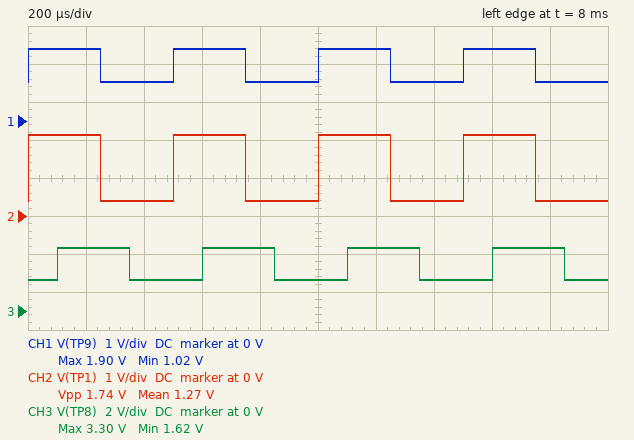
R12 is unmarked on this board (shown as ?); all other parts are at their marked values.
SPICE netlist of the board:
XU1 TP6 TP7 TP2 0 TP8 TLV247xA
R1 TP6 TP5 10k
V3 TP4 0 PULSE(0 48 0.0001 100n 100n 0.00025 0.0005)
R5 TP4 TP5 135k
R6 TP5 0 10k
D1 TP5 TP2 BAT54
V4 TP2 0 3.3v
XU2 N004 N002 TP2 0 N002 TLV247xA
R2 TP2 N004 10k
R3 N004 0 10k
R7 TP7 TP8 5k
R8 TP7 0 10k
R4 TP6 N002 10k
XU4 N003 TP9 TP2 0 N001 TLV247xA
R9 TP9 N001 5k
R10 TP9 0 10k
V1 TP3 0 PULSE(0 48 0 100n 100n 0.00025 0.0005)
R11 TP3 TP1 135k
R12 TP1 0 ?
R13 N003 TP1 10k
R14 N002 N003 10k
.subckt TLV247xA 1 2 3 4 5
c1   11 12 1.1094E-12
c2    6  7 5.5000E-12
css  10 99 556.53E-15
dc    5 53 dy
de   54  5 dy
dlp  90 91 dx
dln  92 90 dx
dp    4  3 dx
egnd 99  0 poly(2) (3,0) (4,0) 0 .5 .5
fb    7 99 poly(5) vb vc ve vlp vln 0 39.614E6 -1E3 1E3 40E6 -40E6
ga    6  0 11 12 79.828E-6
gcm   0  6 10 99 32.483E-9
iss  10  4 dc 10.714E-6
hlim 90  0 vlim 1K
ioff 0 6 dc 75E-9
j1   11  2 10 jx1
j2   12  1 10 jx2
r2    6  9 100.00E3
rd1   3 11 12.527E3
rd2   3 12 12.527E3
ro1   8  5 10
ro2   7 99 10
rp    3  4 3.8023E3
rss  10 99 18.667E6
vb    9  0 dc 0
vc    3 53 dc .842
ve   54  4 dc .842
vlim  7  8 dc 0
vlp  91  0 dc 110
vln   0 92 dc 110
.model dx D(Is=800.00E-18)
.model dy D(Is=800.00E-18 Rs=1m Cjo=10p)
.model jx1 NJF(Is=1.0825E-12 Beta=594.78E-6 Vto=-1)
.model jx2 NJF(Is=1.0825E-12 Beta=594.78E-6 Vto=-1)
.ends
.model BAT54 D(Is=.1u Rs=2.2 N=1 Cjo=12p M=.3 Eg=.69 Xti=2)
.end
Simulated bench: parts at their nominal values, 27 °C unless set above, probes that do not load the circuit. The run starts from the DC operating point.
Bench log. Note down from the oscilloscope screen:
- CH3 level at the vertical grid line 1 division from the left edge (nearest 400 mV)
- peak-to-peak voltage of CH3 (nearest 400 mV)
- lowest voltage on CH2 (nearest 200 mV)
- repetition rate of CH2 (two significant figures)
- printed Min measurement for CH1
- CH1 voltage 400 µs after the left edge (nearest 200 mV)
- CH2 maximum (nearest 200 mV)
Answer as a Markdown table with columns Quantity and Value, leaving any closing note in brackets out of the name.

| Quantity | Value |
|---|---|
| CH3 level at the vertical grid line 1 division from the left edge | 3.2 V |
| peak-to-peak voltage of CH3 | 1.6 V |
| lowest voltage on CH2 | 400 mV |
| repetition rate of CH2 | 2.0 kHz |
| printed Min measurement for CH1 | 1.02 V |
| CH1 voltage 400 µs after the left edge | 1.0 V |
| CH2 maximum | 2.2 V |
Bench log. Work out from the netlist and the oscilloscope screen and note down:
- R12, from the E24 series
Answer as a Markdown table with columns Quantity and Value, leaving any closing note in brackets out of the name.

| Quantity | Value |
|---|---|
| R12, from the E24 series | 6.8 kΩ |
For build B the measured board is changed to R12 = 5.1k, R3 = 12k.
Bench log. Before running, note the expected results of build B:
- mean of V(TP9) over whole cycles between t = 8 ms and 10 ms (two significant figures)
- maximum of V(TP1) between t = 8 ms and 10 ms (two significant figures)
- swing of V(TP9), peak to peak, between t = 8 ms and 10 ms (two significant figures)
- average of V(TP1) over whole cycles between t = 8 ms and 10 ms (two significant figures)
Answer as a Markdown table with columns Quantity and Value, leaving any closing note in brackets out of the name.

| Quantity | Value |
|---|---|
| mean of V(TP9) over whole cycles between t = 8 ms and 10 ms | 1.4 V |
| maximum of V(TP1) between t = 8 ms and 10 ms | 1.8 V |
| swing of V(TP9), peak to peak, between t = 8 ms and 10 ms | 700 mV |
| average of V(TP1) over whole cycles between t = 8 ms and 10 ms | 1.1 V |
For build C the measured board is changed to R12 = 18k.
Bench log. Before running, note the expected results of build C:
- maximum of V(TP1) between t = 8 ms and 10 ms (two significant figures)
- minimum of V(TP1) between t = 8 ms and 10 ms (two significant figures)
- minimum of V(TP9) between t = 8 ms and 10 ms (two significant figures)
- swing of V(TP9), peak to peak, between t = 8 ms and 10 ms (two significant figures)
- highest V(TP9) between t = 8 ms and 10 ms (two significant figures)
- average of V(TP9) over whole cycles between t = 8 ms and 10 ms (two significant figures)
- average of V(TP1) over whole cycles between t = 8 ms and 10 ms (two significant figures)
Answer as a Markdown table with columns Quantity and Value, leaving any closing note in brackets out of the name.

| Quantity | Value |
|---|---|
| maximum of V(TP1) between t = 8 ms and 10 ms | 3.9 V |
| minimum of V(TP1) between t = 8 ms and 10 ms | 730 mV |
| minimum of V(TP9) between t = 8 ms and 10 ms | 1.2 V |
| swing of V(TP9), peak to peak, between t = 8 ms and 10 ms | 1.0 V |
| highest V(TP9) between t = 8 ms and 10 ms | 2.2 V |
| average of V(TP9) over whole cycles between t = 8 ms and 10 ms | 1.7 V |
| average of V(TP1) over whole cycles between t = 8 ms and 10 ms | 2.3 V |
